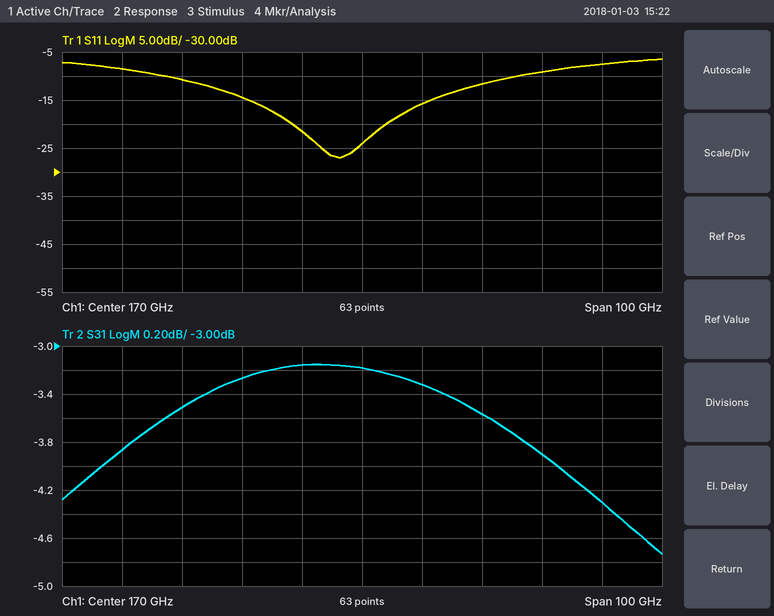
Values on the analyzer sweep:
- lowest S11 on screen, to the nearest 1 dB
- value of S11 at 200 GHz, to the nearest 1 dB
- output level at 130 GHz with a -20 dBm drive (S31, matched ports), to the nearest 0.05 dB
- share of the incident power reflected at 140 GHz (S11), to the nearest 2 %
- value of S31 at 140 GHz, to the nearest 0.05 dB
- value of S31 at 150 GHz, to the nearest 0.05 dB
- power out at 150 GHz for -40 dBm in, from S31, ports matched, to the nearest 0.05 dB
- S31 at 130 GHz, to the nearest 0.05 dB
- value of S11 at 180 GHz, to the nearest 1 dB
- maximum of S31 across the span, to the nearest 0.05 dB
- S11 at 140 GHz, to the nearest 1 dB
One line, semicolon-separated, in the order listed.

-27 dB; -9 dB; -23.85 dBm; 8 %; -3.50 dB; -3.25 dB; -43.25 dBm; -3.85 dB; -16 dB; -3.15 dB; -11 dB
